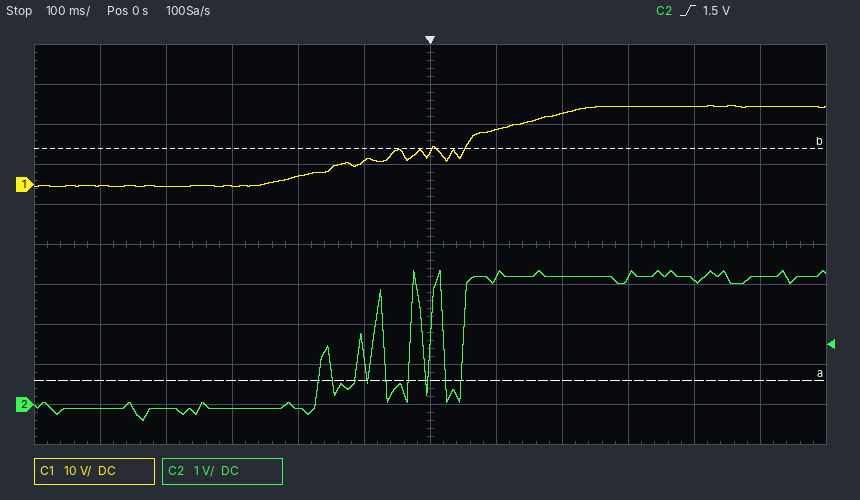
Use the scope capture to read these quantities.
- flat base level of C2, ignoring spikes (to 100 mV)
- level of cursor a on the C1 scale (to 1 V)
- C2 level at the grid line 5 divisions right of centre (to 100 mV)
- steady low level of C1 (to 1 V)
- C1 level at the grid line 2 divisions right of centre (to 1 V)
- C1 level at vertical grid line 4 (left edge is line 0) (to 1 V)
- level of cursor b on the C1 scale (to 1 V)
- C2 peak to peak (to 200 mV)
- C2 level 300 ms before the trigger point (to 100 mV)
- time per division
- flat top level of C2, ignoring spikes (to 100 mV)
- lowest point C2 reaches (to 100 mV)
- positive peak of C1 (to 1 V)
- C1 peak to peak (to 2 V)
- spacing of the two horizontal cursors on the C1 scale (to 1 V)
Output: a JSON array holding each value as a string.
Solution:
["-100 mV", "-49 V", "3.2 V", "0 V", "18 V", "2 V", "9 V", "3.8 V", "-100 mV", "100 ms", "3.2 V", "-400 mV", "20 V", "20 V", "58 V"]
